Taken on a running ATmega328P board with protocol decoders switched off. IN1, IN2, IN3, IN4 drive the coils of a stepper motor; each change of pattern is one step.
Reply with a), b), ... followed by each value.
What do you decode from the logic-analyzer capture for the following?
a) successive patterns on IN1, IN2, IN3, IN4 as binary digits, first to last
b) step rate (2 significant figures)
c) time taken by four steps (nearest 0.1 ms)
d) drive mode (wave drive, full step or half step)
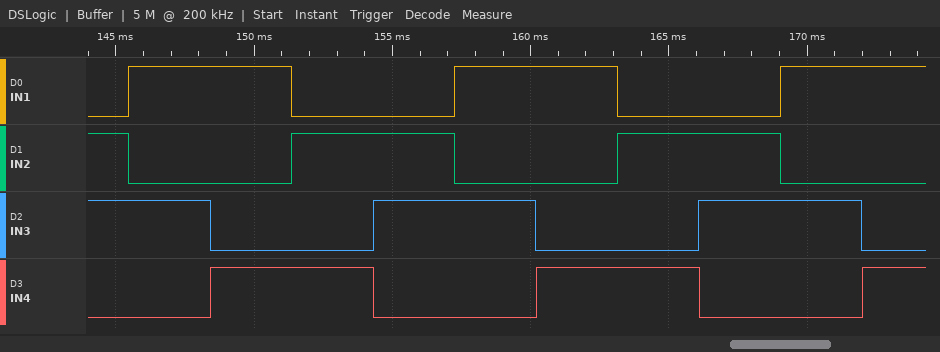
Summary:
a) 0110 1010 1001 0101 0110 1010 1001 0101 0110 1010 1001
b) 340 steps/s
c) 11.8 ms
d) full step
